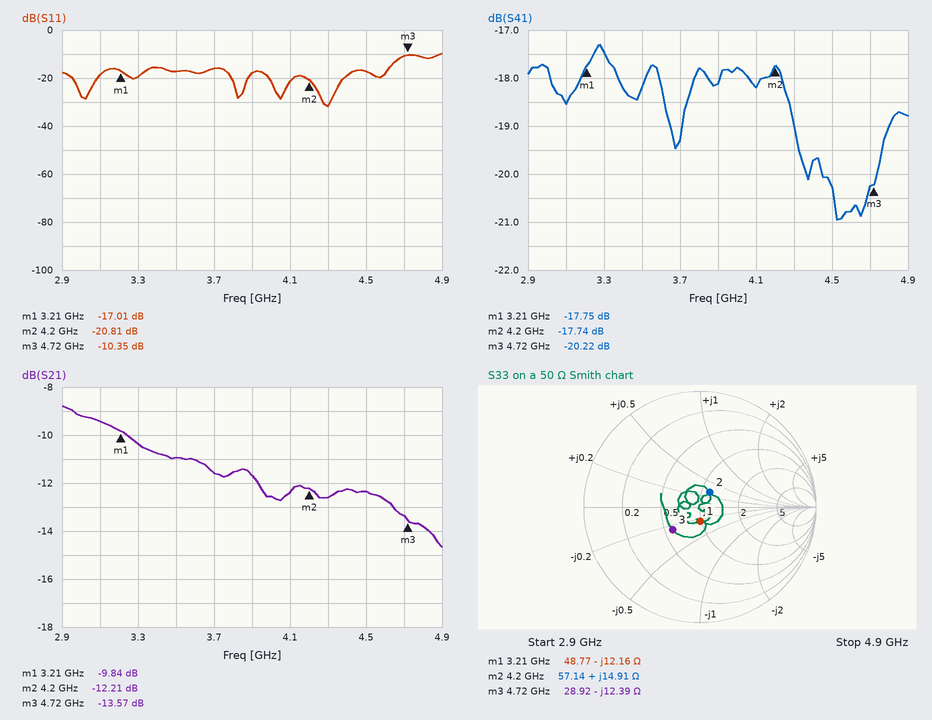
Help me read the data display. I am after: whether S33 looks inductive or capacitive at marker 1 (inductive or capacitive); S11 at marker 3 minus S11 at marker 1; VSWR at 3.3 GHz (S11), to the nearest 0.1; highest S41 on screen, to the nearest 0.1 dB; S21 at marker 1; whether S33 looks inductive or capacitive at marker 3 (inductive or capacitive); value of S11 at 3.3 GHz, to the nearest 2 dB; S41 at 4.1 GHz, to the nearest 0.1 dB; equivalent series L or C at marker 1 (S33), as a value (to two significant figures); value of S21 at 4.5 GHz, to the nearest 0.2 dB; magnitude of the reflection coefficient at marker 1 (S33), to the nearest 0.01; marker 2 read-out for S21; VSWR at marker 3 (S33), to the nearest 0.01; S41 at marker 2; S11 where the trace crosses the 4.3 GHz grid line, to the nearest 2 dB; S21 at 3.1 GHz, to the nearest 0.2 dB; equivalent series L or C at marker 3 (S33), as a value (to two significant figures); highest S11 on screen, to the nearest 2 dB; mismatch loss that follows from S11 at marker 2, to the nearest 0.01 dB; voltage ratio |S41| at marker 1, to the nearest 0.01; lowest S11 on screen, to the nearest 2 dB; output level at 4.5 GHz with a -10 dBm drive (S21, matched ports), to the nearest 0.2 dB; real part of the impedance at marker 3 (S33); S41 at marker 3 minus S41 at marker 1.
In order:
capacitive
6.66 dB
1.2
-17.3 dB
-9.84 dB
capacitive
-20 dB
-18.2 dB
4.1 pF
-12.4 dB
0.12
-12.21 dB
1.88
-17.74 dB
-32 dB
-9.4 dB
2.7 pF
-10 dB
0.04 dB
0.13
-32 dB
-22.4 dBm
28.92 Ω
-2.47 dB
